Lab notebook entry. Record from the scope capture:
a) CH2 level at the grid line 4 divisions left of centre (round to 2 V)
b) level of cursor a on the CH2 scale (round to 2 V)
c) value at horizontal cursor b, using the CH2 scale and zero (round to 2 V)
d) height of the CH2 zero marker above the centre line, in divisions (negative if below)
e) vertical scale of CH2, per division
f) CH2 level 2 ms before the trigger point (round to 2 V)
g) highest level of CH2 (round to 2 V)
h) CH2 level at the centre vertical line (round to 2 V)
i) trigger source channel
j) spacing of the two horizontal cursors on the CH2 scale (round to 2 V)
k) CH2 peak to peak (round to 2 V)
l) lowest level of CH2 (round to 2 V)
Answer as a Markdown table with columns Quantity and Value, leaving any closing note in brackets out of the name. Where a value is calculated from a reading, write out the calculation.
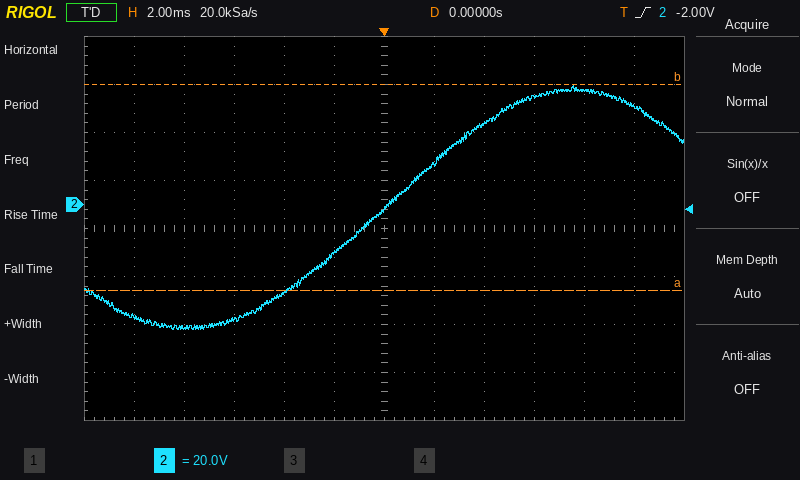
| Quantity | Value |
|---|---|
| CH2 level at the grid line 4 divisions left of centre | -52 V |
| level of cursor a on the CH2 scale | -36 V |
| value at horizontal cursor b, using the CH2 scale and zero | 50 V |
| height of the CH2 zero marker above the centre line, in divisions | +0.5 div |
| vertical scale of CH2, per division | 20 V |
| CH2 level 2 ms before the trigger point | -20 V |
| highest level of CH2 | 50 V |
| CH2 level at the centre vertical line | -2 V |
| trigger source channel | CH2 |
| spacing of the two horizontal cursors on the CH2 scale | 86 V |
| CH2 peak to peak | 50 V − (-52 V) = 102 V |
| lowest level of CH2 | -52 V |
